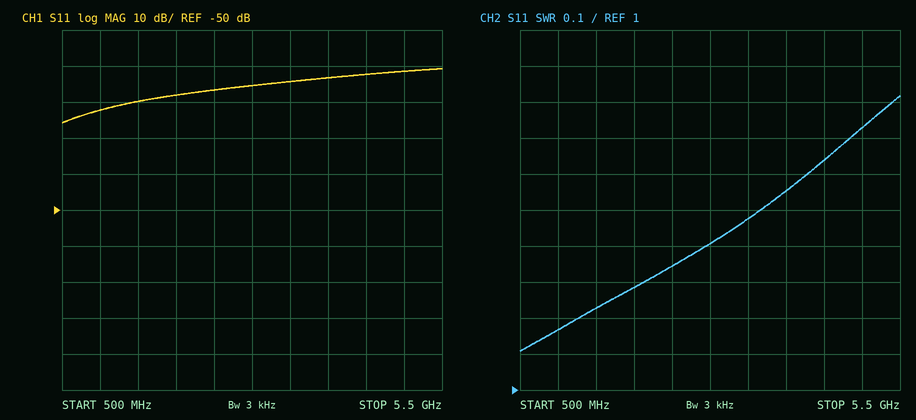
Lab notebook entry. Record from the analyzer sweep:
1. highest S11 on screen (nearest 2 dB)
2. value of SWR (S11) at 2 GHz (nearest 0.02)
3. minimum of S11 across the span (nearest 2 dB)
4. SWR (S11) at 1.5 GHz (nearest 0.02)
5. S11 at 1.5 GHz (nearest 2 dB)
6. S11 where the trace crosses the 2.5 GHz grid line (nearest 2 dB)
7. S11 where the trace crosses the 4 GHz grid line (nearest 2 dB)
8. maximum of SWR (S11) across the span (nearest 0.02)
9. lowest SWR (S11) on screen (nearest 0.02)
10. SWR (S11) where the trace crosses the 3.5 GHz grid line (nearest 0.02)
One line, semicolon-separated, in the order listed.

-10 dB; 1.28; -26 dB; 1.22; -20 dB; -16 dB; -14 dB; 1.82; 1.10; 1.48
